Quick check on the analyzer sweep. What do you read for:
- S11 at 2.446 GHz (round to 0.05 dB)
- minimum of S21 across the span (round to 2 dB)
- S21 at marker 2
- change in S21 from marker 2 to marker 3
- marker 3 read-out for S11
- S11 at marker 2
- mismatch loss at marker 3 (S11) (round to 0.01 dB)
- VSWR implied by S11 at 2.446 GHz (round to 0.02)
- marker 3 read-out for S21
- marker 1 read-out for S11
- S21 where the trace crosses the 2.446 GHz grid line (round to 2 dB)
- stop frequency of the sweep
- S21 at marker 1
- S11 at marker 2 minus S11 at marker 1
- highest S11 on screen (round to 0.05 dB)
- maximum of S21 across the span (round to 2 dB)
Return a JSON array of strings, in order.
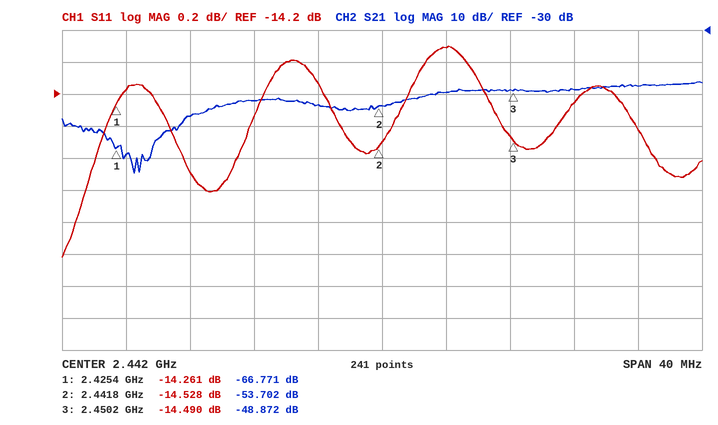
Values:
["-13.90 dB", "-74 dB", "-53.702 dB", "4.830 dB", "-14.490 dB", "-14.528 dB", "0.16 dB", "1.50", "-48.872 dB", "-14.261 dB", "-50 dB", "2.462 GHz", "-66.771 dB", "-0.267 dB", "-13.90 dB", "-46 dB"]
